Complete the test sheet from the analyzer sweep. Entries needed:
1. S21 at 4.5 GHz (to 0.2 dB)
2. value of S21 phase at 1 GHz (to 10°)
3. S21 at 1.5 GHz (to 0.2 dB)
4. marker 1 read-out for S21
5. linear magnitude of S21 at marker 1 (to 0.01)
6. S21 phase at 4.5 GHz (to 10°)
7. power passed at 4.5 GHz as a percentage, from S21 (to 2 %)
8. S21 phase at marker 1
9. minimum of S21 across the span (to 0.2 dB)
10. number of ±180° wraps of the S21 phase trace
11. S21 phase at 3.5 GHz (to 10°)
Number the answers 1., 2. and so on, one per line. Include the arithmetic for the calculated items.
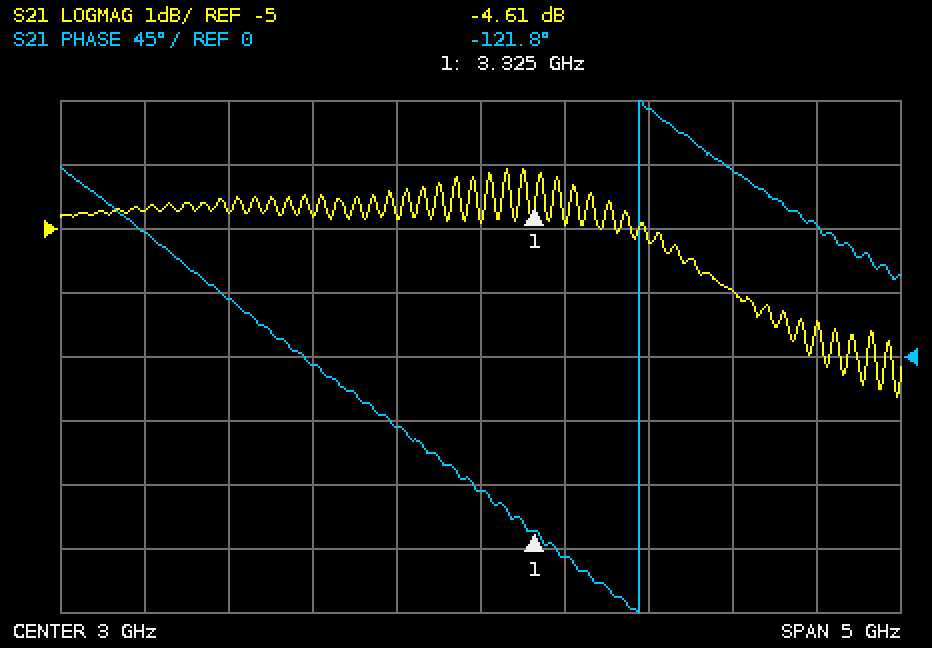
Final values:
1. -6.0 dB
2. 90°
3. -4.8 dB
4. -4.61 dB
5. 10^(-4.61/20) ≈ 0.59
6. 130°
7. 10^(-6/10) ≈ 25.1 %, so 26 % to the nearest 2 %
8. -121.8°
9. -7.6 dB
10. 1
11. -140°
